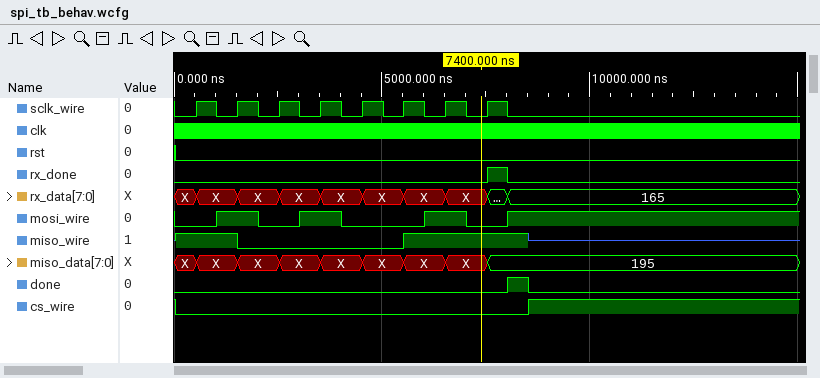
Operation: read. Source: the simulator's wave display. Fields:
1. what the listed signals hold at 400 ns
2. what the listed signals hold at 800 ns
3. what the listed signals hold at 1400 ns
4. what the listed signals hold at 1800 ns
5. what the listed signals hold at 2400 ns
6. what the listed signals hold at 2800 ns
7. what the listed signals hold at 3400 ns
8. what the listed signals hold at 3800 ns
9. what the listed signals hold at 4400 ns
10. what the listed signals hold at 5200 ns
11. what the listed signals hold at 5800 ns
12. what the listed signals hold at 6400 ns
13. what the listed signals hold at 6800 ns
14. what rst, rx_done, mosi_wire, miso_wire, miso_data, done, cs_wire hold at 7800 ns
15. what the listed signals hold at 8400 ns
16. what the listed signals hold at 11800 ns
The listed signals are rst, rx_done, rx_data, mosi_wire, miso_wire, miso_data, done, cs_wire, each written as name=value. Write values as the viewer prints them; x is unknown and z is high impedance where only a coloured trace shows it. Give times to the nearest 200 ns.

rst=0, rx_done=0, rx_data=X, mosi_wire=0, miso_wire=1, miso_data=X, done=0, cs_wire=0
rst=0, rx_done=0, rx_data=X, mosi_wire=0, miso_wire=1, miso_data=X, done=0, cs_wire=0
rst=0, rx_done=0, rx_data=X, mosi_wire=1, miso_wire=1, miso_data=X, done=0, cs_wire=0
rst=0, rx_done=0, rx_data=X, mosi_wire=1, miso_wire=0, miso_data=X, done=0, cs_wire=0
rst=0, rx_done=0, rx_data=X, mosi_wire=0, miso_wire=0, miso_data=X, done=0, cs_wire=0
rst=0, rx_done=0, rx_data=X, mosi_wire=0, miso_wire=0, miso_data=X, done=0, cs_wire=0
rst=0, rx_done=0, rx_data=X, mosi_wire=1, miso_wire=0, miso_data=X, done=0, cs_wire=0
rst=0, rx_done=0, rx_data=X, mosi_wire=1, miso_wire=0, miso_data=X, done=0, cs_wire=0
rst=0, rx_done=0, rx_data=X, mosi_wire=0, miso_wire=0, miso_data=X, done=0, cs_wire=0
rst=0, rx_done=0, rx_data=X, mosi_wire=0, miso_wire=0, miso_data=X, done=0, cs_wire=0
rst=0, rx_done=0, rx_data=X, mosi_wire=0, miso_wire=1, miso_data=X, done=0, cs_wire=0
rst=0, rx_done=0, rx_data=X, mosi_wire=1, miso_wire=1, miso_data=X, done=0, cs_wire=0
rst=0, rx_done=0, rx_data=X, mosi_wire=1, miso_wire=1, miso_data=X, done=0, cs_wire=0
rst=0, rx_done=1, mosi_wire=0, miso_wire=1, miso_data=195, done=0, cs_wire=0
rst=0, rx_done=0, rx_data=165, mosi_wire=1, miso_wire=1, miso_data=195, done=1, cs_wire=0
rst=0, rx_done=0, rx_data=165, mosi_wire=1, miso_wire=z, miso_data=195, done=0, cs_wire=1
